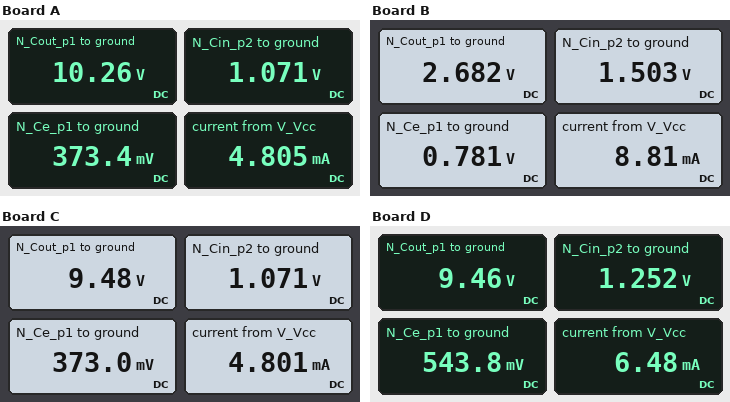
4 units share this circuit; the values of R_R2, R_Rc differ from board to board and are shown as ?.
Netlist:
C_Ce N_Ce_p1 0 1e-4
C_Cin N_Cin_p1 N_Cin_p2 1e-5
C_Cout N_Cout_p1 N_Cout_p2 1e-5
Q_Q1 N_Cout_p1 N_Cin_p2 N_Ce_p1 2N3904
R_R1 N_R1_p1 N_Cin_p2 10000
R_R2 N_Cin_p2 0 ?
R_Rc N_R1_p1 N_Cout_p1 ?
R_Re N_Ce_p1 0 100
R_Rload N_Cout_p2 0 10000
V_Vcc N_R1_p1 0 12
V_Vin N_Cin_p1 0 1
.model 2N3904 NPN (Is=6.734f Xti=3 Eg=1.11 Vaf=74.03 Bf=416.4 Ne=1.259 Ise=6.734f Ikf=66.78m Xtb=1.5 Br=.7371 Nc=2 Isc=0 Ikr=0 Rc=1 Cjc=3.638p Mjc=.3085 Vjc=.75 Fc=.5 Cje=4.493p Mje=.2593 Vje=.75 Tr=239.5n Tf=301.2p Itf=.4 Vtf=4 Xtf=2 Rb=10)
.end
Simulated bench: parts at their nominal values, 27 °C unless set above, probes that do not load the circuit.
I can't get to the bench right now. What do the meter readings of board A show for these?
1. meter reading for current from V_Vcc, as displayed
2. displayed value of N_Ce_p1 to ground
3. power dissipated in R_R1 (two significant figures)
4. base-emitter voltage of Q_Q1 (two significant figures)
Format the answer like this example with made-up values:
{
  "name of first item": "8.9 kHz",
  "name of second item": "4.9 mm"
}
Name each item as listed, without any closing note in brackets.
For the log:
{
  "meter reading for current from V_Vcc, as displayed": "4.805 mA",
  "displayed value of N_Ce_p1 to ground": "373.4 mV",
  "power dissipated in R_R1": "12 mW",
  "base-emitter voltage of Q_Q1": "700 mV"
}
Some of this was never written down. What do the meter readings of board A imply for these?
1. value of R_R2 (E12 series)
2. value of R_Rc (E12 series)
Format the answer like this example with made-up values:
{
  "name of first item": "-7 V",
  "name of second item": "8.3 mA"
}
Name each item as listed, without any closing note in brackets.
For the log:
{
  "value of R_R2": "1 kΩ",
  "value of R_Rc": "470 Ω"
}
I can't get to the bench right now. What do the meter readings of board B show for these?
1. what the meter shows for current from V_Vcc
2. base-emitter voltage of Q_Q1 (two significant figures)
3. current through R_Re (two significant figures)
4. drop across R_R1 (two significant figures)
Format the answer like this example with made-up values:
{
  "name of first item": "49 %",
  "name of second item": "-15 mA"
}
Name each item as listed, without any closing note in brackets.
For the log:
{
  "what the meter shows for current from V_Vcc": "8.81 mA",
  "base-emitter voltage of Q_Q1": "720 mV",
  "current through R_Re": "7.8 mA",
  "drop across R_R1": "10 V"
}
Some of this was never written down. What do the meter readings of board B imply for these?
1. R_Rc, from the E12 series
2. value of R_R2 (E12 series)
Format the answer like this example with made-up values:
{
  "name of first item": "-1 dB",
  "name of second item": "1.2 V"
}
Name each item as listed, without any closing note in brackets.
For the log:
{
  "R_Rc, from the E12 series": "1.2 kΩ",
  "value of R_R2": "1.5 kΩ"
}
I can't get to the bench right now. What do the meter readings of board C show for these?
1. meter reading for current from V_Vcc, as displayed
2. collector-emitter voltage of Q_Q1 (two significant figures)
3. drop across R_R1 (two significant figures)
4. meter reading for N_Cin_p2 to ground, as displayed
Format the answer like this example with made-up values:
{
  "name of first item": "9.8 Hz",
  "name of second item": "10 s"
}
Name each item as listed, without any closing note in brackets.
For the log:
{
  "meter reading for current from V_Vcc, as displayed": "4.801 mA",
  "collector-emitter voltage of Q_Q1": "9.1 V",
  "drop across R_R1": "11 V",
  "meter reading for N_Cin_p2 to ground, as displayed": "1.071 V"
}
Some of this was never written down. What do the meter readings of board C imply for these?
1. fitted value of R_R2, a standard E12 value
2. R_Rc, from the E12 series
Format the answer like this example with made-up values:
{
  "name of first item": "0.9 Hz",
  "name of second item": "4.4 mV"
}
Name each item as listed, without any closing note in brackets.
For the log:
{
  "fitted value of R_R2, a standard E12 value": "1 kΩ",
  "R_Rc, from the E12 series": "680 Ω"
}
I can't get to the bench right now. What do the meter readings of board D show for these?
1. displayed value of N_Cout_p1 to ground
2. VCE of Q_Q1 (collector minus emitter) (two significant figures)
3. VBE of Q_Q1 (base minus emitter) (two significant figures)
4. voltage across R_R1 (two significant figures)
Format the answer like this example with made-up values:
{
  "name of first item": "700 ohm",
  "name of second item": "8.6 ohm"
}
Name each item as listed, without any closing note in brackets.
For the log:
{
  "displayed value of N_Cout_p1 to ground": "9.46 V",
  "VCE of Q_Q1 (collector minus emitter)": "8.9 V",
  "VBE of Q_Q1 (base minus emitter)": "710 mV",
  "voltage across R_R1": "11 V"
}
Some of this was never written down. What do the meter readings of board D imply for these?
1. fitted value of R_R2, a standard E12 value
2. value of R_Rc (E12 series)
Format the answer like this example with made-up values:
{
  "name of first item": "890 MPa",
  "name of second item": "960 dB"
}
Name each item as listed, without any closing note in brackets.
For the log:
{
  "fitted value of R_R2, a standard E12 value": "1.2 kΩ",
  "value of R_Rc": "470 Ω"
}
